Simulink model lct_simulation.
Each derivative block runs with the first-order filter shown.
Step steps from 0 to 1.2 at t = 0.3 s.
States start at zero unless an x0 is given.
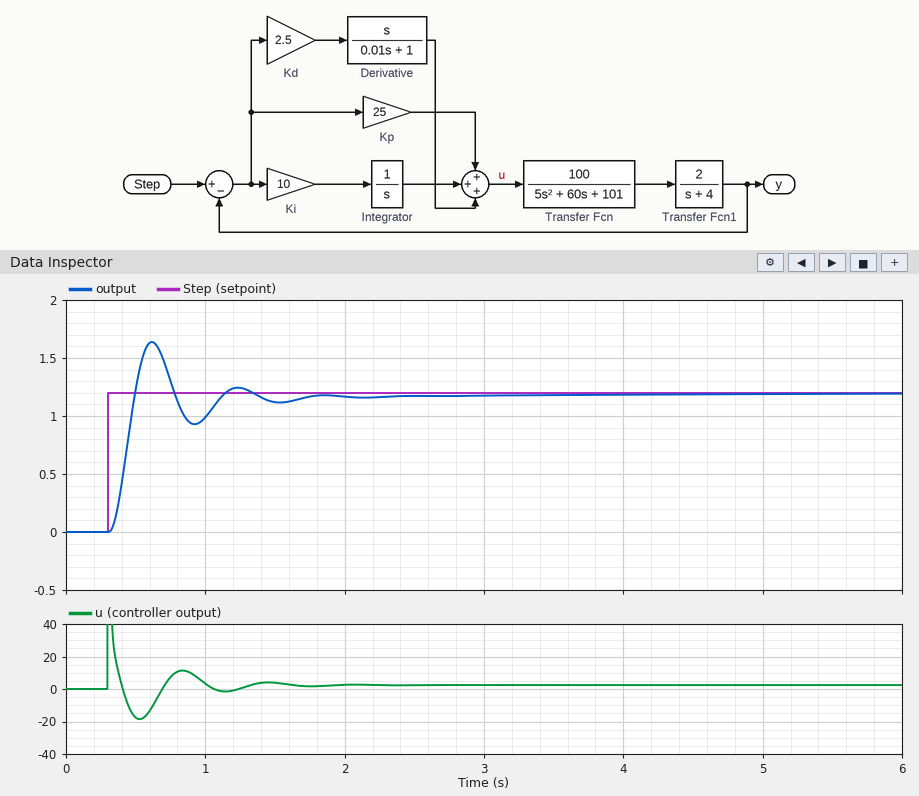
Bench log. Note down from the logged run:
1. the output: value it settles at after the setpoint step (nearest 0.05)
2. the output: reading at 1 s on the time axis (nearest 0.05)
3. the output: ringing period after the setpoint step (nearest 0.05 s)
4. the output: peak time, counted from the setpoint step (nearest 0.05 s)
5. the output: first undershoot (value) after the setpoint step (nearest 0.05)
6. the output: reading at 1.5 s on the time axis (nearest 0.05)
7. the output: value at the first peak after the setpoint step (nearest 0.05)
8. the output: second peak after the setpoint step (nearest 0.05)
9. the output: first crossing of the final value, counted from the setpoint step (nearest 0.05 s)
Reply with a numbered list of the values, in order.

1. 1.20
2. 1.00
3. 0.60 s
4. 0.30 s
5. 0.95
6. 1.10
7. 1.65
8. 1.25
9. 0.20 s
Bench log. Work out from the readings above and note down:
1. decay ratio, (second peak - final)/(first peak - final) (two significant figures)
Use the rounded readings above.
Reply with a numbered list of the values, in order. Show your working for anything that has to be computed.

1. (1.25 - 1.2) / (1.65 - 1.2) = 0.11
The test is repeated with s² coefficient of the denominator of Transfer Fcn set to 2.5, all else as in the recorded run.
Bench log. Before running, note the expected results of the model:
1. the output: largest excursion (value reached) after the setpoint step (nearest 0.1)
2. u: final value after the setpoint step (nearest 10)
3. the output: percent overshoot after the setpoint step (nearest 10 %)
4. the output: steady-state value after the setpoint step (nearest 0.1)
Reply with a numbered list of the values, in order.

1. 1.4
2. 0
3. 20 %
4. 1.2
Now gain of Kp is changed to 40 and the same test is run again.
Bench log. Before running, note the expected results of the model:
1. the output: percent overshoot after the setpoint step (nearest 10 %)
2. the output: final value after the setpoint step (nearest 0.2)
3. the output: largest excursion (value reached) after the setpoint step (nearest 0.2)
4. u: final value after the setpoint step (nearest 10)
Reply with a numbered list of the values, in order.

1. 60 %
2. 1.2
3. 2.0
4. 0
